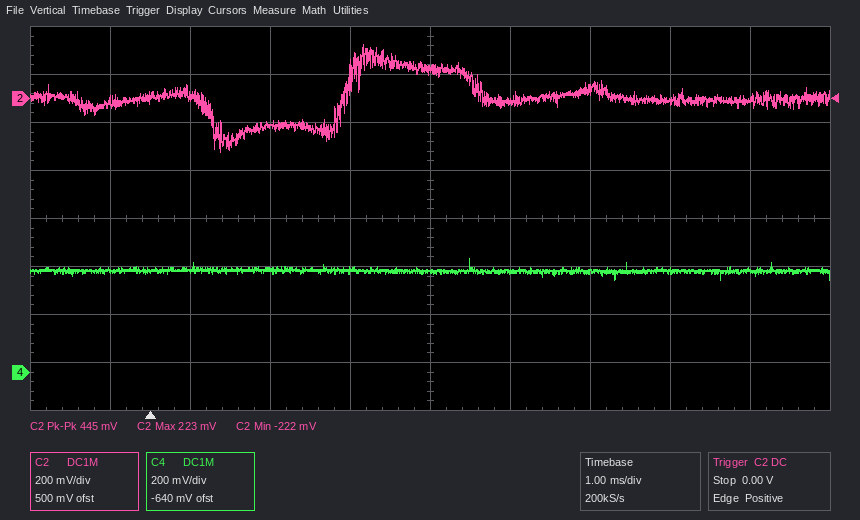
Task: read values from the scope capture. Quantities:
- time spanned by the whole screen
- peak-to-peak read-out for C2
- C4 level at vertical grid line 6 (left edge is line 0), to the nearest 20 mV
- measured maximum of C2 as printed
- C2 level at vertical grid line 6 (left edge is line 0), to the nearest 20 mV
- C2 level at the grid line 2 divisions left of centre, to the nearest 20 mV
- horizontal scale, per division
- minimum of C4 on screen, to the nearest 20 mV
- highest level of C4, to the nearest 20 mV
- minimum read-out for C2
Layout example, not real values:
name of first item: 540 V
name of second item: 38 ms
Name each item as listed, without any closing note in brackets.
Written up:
time spanned by the whole screen: 10 ms
peak-to-peak read-out for C2: 445 mV
C4 level at vertical grid line 6 (left edge is line 0), to the nearest 20 mV: 420 mV
measured maximum of C2 as printed: 223 mV
C2 level at vertical grid line 6 (left edge is line 0), to the nearest 20 mV: 0 mV
C2 level at the grid line 2 divisions left of centre, to the nearest 20 mV: -100 mV
horizontal scale, per division: 1 ms
minimum of C4 on screen, to the nearest 20 mV: 380 mV
highest level of C4, to the nearest 20 mV: 480 mV
minimum read-out for C2: -222 mV
